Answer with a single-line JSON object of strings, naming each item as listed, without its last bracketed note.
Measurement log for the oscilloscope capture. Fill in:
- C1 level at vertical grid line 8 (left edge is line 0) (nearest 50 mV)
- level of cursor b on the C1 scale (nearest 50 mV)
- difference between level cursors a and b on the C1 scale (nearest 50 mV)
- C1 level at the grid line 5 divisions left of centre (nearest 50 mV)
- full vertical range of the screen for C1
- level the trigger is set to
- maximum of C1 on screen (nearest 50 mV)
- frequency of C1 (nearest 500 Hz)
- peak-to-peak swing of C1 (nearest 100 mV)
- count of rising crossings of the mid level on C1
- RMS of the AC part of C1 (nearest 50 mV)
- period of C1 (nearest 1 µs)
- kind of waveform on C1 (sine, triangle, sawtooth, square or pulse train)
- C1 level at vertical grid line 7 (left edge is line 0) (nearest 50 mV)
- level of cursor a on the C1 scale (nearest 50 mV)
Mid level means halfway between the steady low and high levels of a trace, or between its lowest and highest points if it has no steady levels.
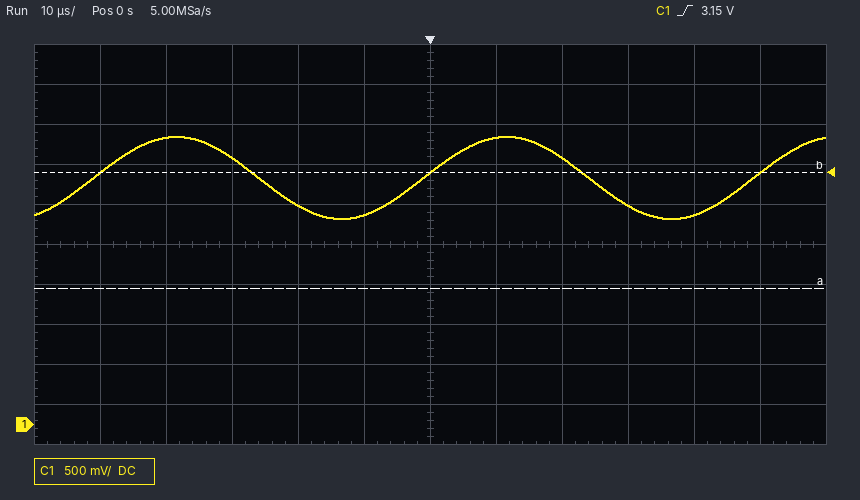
{"C1 level at vertical grid line 8 (left edge is line 0)": "3.35 V", "level of cursor b on the C1 scale": "3.15 V", "difference between level cursors a and b on the C1 scale": "1.45 V", "C1 level at the grid line 5 divisions left of centre": "3.15 V", "full vertical range of the screen for C1": "5 V", "level the trigger is set to": "3.15 V", "maximum of C1 on screen": "3.60 V", "frequency of C1": "20.0 kHz", "peak-to-peak swing of C1": "1.00 V", "count of rising crossings of the mid level on C1": "3", "RMS of the AC part of C1": "350 mV", "period of C1": "50 µs", "kind of waveform on C1": "sine", "C1 level at vertical grid line 7 (left edge is line 0)": "3.60 V", "level of cursor a on the C1 scale": "1.70 V"}
